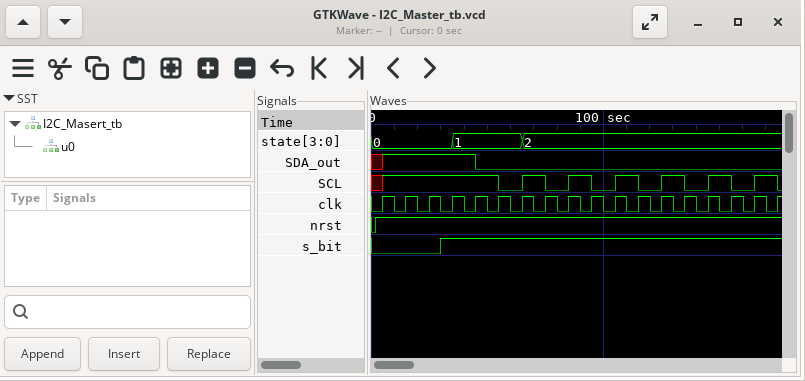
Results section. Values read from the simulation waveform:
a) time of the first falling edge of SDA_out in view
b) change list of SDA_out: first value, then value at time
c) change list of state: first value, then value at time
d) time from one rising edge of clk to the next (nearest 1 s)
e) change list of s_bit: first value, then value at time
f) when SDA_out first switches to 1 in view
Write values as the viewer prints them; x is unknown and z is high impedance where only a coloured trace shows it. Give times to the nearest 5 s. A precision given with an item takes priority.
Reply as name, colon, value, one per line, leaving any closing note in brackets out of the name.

time of the first falling edge of SDA_out in view: 45 s
change list of SDA_out: first value, then value at time: x, 1 at 5 s, 0 at 45 s
change list of state: first value, then value at time: 0, 1 at 35 s, 2 at 65 s
time from one rising edge of clk to the next: 10 s
change list of s_bit: first value, then value at time: 0, 1 at 30 s
when SDA_out first switches to 1 in view: 5 s
